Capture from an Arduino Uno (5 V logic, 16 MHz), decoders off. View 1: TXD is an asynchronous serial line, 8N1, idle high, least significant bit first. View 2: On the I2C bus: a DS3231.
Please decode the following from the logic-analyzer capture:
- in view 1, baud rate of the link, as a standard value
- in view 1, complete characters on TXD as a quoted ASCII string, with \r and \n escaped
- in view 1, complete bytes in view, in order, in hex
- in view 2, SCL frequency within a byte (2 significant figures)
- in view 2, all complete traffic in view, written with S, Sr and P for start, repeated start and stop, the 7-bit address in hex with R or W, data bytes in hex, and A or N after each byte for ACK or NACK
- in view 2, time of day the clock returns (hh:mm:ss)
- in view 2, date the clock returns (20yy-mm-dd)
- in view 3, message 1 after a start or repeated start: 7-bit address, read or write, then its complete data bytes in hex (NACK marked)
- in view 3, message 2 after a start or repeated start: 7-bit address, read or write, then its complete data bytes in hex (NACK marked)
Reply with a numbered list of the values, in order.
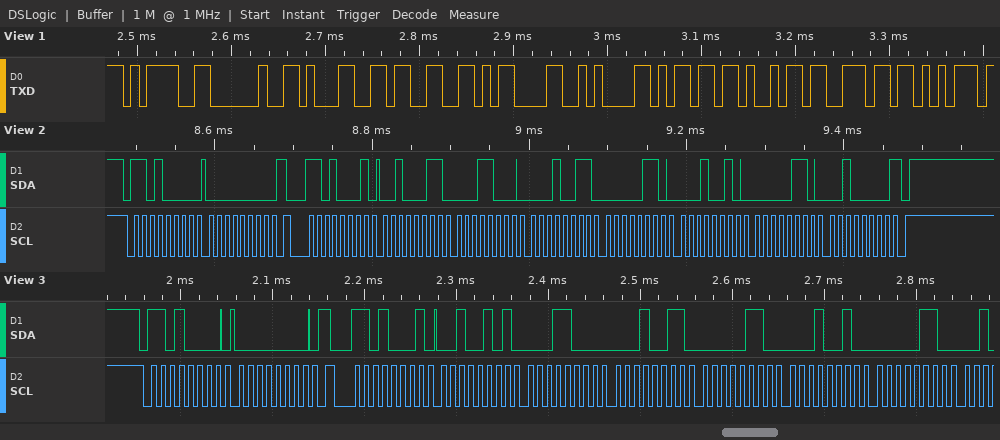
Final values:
1. 115200 baud
2. "= 13\r\nminu"
3. 0x3D 0x20 0x31 0x33 0x0D 0x0A 0x6D 0x69 0x6E 0x75
4. 100 kHz
5. S 68W A 00 A Sr 68R A 23 A 18 A 13 A 06 A 12 A 06 A 20 N P
6. 13:18:23
7. 2020-06-12
8. 0x68 write: 00
9. 0x68 read: 25 18 13 06 12 06
